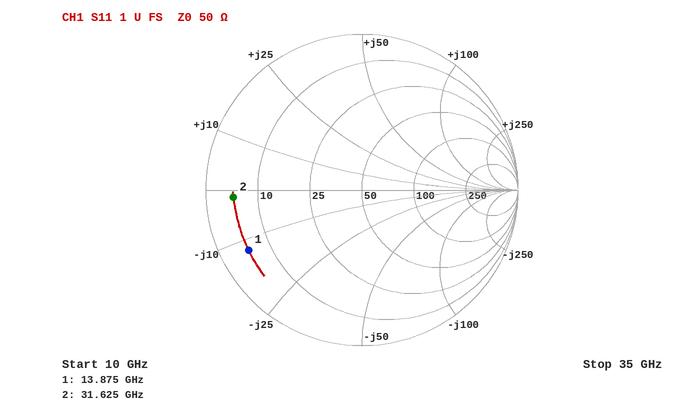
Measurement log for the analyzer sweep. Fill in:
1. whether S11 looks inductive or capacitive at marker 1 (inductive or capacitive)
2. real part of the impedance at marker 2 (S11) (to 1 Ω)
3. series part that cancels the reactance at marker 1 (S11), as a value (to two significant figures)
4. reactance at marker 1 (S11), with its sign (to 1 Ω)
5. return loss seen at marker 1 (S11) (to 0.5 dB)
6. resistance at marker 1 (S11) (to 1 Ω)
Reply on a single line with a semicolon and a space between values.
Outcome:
capacitive; 5 Ω; 140 pH; -12 Ω; 1.5 dB; 5 Ω
